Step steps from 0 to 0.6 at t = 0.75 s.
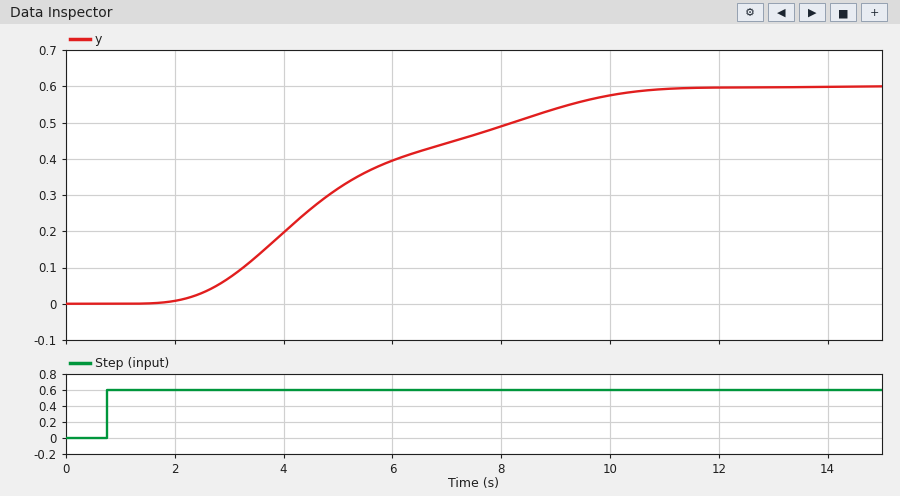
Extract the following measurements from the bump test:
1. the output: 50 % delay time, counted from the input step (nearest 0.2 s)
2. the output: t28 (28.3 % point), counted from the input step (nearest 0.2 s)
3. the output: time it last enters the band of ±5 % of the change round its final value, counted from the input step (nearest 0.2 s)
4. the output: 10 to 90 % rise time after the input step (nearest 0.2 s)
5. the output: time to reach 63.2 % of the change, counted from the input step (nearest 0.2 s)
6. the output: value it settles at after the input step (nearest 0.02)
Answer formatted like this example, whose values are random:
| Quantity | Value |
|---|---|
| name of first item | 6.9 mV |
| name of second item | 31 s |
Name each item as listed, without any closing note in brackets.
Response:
| Quantity | Value |
|---|---|
| the output: 50 % delay time, counted from the input step | 4.0 s |
| the output: t28 (28.3 % point), counted from the input step | 3.0 s |
| the output: time it last enters the band of ±5 % of the change round its final value, counted from the input step | 9.0 s |
| the output: 10 to 90 % rise time after the input step | 6.2 s |
| the output: time to reach 63.2 % of the change, counted from the input step | 5.0 s |
| the output: value it settles at after the input step | 0.60 |
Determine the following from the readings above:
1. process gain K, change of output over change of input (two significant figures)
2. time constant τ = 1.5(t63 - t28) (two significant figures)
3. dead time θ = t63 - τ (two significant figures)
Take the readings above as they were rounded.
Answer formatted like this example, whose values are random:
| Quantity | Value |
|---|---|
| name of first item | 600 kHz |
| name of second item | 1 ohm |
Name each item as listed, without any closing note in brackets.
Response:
| Quantity | Value |
|---|---|
| process gain K, change of output over change of input | 1.0 |
| time constant τ = 1.5(t63 - t28) | 3.0 s |
| dead time θ = t63 - τ | 2.0 s |
